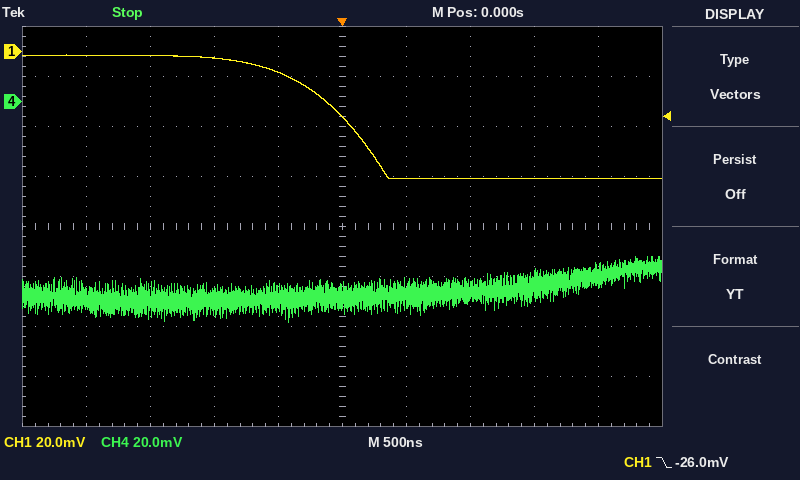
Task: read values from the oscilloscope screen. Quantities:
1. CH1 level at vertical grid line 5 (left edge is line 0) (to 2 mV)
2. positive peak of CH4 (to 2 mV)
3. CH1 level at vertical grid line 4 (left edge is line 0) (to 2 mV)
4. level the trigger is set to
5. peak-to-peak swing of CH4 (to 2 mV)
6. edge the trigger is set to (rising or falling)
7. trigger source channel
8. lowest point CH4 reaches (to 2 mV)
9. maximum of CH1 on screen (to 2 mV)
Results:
-26 mV
-62 mV
-8 mV
-26.0 mV
26 mV
falling
CH1
-88 mV
-2 mV
